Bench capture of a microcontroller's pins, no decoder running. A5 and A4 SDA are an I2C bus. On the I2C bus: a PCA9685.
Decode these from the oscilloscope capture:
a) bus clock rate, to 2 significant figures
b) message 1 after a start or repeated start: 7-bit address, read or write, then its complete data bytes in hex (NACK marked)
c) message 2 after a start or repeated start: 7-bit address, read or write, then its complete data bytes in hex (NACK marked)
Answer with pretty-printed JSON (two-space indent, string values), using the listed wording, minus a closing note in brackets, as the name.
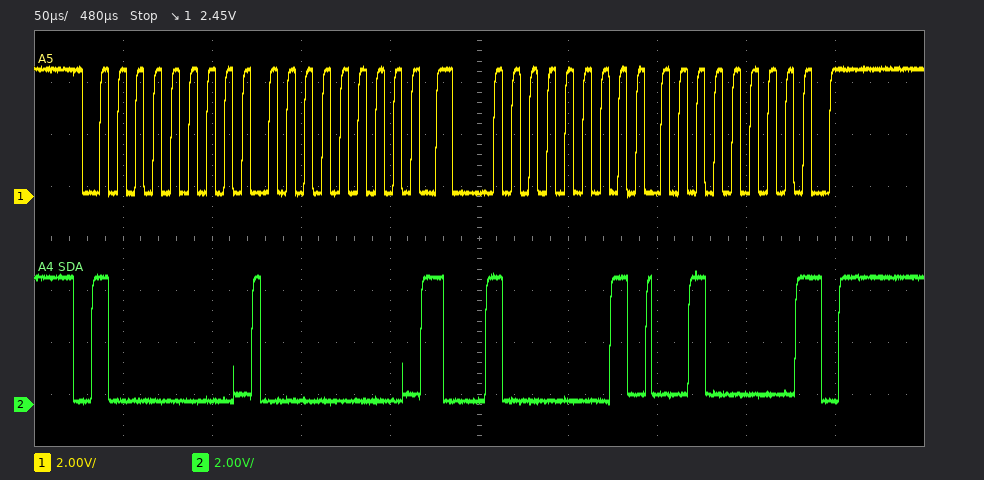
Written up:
{
  "bus clock rate, to 2 significant figures": "100 kHz",
  "message 1 after a start or repeated start: 7-bit address, read or write, then its complete data bytes in hex": "0x40 write: 00",
  "message 2 after a start or repeated start: 7-bit address, read or write, then its complete data bytes in hex": "0x40 read: 20 NACK"
}
